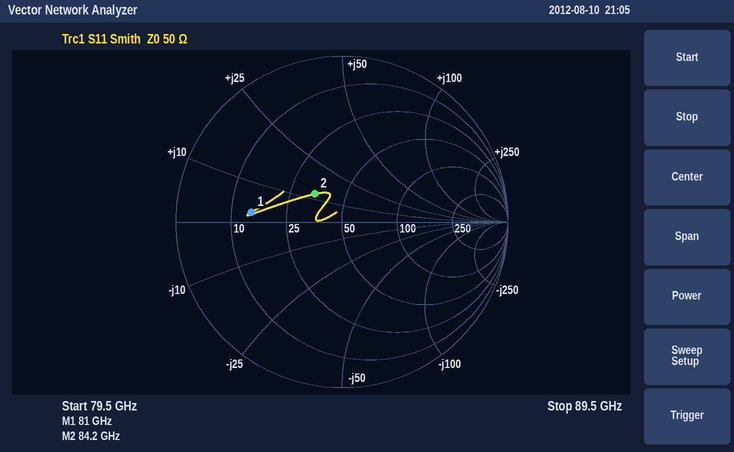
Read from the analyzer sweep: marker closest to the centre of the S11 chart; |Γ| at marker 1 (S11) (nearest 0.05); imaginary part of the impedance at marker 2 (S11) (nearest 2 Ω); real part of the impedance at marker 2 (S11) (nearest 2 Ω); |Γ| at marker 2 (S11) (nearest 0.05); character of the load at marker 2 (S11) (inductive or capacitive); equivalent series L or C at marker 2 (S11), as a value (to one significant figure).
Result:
marker 2
0.55
+12 Ω
34 Ω
0.25
inductive
20 pH
